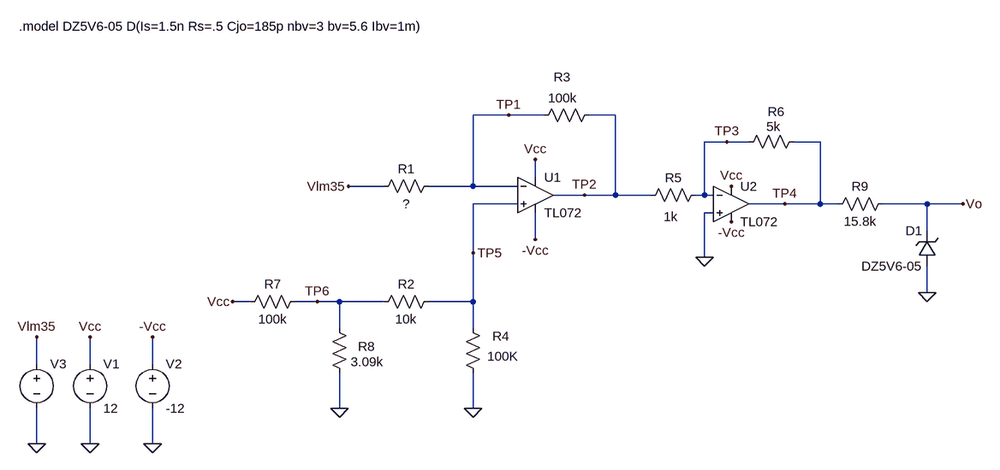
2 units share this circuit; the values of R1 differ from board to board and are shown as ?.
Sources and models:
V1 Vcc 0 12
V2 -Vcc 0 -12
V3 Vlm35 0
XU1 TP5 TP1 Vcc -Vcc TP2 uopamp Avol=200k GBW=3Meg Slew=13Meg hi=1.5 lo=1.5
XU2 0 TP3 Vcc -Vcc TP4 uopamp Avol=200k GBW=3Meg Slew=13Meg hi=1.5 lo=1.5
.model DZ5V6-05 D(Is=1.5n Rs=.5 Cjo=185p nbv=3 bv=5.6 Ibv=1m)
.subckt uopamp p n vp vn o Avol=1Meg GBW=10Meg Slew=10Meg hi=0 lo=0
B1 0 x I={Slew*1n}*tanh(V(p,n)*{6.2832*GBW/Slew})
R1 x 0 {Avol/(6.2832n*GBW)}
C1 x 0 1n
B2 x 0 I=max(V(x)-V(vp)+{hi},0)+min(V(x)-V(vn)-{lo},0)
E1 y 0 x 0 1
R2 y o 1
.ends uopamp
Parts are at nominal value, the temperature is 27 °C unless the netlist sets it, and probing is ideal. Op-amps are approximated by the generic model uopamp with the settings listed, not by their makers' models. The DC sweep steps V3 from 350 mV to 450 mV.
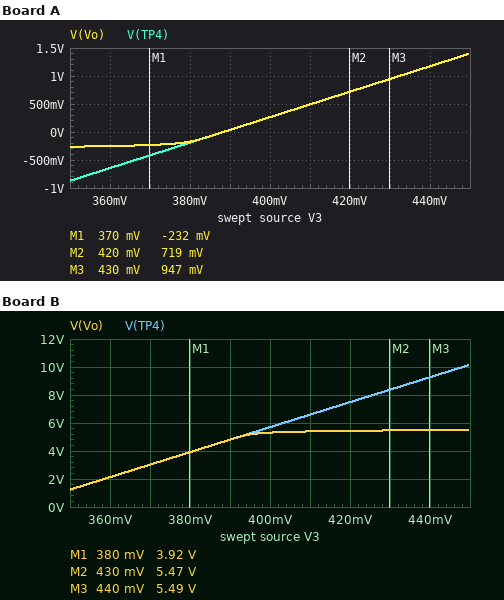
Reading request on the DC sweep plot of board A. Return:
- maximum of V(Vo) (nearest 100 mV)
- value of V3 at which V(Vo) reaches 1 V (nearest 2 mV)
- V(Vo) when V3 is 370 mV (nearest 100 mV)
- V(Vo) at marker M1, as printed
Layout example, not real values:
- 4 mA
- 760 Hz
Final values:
- 1.4 V
- 432 mV
- -200 mV
- -232 mV
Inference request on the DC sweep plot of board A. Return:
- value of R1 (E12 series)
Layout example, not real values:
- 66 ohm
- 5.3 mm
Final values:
- 22 kΩ
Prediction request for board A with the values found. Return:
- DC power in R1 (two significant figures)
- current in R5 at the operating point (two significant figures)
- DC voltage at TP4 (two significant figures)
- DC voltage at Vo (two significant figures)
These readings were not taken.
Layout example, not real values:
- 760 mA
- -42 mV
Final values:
- 4.6 µW
- 1.8 mA
- -8.8 V
- -330 mV
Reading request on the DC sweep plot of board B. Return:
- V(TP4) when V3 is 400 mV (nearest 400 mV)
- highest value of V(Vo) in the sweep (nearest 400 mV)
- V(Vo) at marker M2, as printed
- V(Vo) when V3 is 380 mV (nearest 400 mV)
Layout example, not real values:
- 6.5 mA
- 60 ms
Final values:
- 5.6 V
- 5.6 V
- 5.47 V
- 4.0 V
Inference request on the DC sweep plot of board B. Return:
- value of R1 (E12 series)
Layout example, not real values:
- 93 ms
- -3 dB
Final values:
- 5.6 kΩ
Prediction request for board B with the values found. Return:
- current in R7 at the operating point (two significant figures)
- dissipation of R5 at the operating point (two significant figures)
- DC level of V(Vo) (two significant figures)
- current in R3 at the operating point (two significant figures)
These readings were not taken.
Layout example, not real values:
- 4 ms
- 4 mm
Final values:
- 120 µA
- 7.6 mW
- -340 mV
- 57 µA
